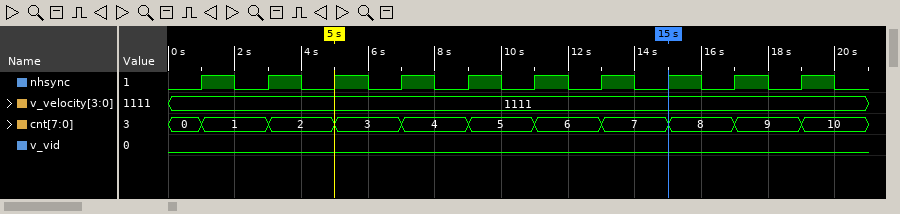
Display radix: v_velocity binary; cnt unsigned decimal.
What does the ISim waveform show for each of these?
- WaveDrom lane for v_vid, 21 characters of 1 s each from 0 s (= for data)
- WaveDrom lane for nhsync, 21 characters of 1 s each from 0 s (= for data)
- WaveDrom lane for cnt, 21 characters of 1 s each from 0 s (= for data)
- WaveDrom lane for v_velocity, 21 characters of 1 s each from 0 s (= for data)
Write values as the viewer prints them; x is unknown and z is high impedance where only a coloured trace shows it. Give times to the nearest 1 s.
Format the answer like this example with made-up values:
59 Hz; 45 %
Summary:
{name: 'v_vid', wave: '0....................'}; {name: 'nhsync', wave: '010101010101010101010'}; {name: 'cnt', wave: '==.=.=.=.=.=.=.=.=.=.', data: '0 1 2 3 4 5 6 7 8 9 10'}; {name: 'v_velocity', wave: '=....................', data: '1111'}
